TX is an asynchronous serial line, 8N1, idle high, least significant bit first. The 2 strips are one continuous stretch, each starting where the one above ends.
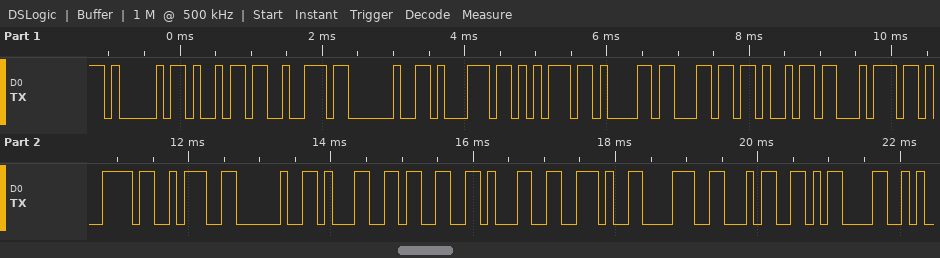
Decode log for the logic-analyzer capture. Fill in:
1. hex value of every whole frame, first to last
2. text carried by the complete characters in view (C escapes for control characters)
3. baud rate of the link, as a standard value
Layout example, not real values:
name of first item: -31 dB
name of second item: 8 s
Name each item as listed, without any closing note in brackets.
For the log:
hex value of every whole frame, first to last: 0x41 0x69 0x72 0x20 0x71 0x75 0x61 0x6C 0x69 0x74 0x79 0x3A 0x20 0x31 0x33 0x31 0x2E 0x38 0x34 0x0D
text carried by the complete characters in view: "Air quality: 131.84\r"
baud rate of the link, as a standard value: 9600 baud
